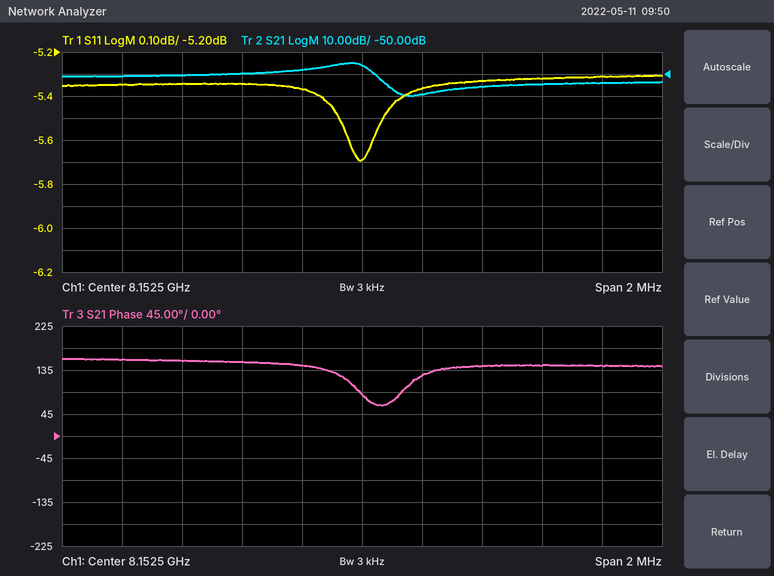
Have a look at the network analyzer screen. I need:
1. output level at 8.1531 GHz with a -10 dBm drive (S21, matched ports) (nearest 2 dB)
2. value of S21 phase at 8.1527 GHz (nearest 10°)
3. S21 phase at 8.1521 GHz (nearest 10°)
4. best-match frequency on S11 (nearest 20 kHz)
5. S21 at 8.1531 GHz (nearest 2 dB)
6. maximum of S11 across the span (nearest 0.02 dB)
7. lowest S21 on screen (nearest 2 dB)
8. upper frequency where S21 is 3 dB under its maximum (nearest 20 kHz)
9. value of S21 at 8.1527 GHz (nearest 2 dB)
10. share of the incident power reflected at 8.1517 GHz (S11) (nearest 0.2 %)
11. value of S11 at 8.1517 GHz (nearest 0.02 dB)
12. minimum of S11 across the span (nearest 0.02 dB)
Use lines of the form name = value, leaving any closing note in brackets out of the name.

output level at 8.1531 GHz with a -10 dBm drive (S21, matched ports) = -64 dBm
value of S21 phase at 8.1527 GHz = 120°
S21 phase at 8.1521 GHz = 150°
best-match frequency on S11 = 8.15250 GHz
S21 at 8.1531 GHz = -54 dB
maximum of S11 across the span = -5.30 dB
lowest S21 on screen = -60 dB
upper frequency where S21 is 3 dB under its maximum = 8.15252 GHz
value of S21 at 8.1527 GHz = -60 dB
share of the incident power reflected at 8.1517 GHz (S11) = 29.2 %
value of S11 at 8.1517 GHz = -5.34 dB
minimum of S11 across the span = -5.70 dB
